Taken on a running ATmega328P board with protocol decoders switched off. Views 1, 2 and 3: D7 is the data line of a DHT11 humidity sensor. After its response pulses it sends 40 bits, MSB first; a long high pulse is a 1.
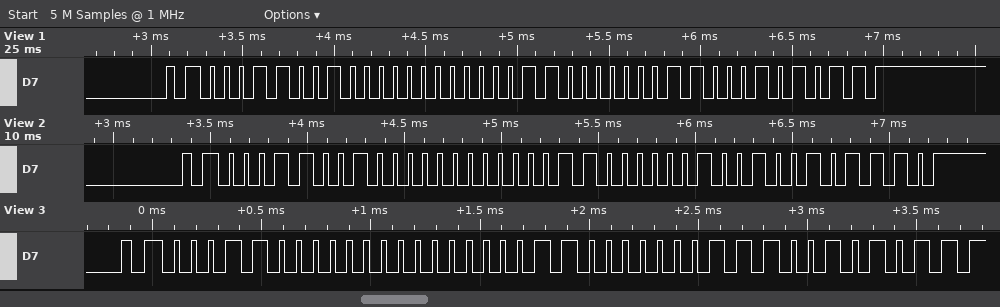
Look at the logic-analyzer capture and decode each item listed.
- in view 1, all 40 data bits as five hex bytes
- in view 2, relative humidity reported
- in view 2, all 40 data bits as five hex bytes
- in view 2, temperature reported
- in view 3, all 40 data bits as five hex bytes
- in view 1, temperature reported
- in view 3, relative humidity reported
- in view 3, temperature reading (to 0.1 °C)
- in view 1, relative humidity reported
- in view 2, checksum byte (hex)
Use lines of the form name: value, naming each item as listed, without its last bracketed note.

in view 1, all 40 data bits as five hex bytes: 19 00 0C 06 2B
in view 2, relative humidity reported: 25 %
in view 2, all 40 data bits as five hex bytes: 19 00 0C 09 2E
in view 2, temperature reported: 12.9 °C
in view 3, all 40 data bits as five hex bytes: 18 00 0C 07 2B
in view 1, temperature reported: 12.6 °C
in view 3, relative humidity reported: 24 %
in view 3, temperature reading: 12.7 °C
in view 1, relative humidity reported: 25 %
in view 2, checksum byte: 0x2E
